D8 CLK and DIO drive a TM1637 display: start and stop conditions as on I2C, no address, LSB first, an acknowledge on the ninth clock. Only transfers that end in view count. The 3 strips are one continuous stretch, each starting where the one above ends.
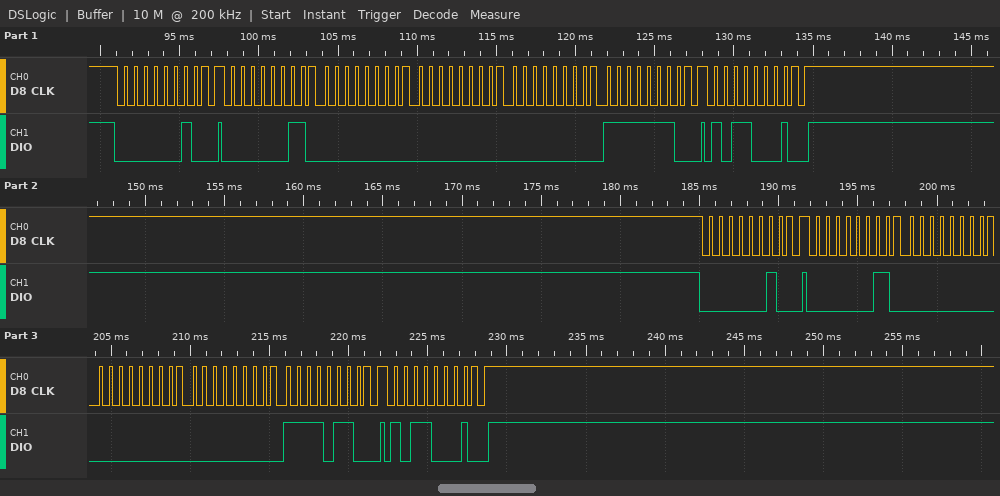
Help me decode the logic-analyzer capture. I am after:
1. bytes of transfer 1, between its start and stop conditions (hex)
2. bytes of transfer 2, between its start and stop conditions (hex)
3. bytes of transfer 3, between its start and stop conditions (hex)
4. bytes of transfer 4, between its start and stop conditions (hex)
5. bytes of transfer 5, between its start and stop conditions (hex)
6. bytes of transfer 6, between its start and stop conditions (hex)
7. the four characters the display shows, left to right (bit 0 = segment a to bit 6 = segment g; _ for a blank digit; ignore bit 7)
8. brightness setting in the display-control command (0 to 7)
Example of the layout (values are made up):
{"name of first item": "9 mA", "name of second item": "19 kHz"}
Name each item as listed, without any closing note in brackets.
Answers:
{"bytes of transfer 1, between its start and stop conditions": "40", "bytes of transfer 2, between its start and stop conditions": "C0 00 00 00 7F", "bytes of transfer 3, between its start and stop conditions": "8D", "bytes of transfer 4, between its start and stop conditions": "40", "bytes of transfer 5, between its start and stop conditions": "C0 00 00 00 6F", "bytes of transfer 6, between its start and stop conditions": "8D", "the four characters the display shows, left to right": "___9", "brightness setting in the display-control command": "5"}
